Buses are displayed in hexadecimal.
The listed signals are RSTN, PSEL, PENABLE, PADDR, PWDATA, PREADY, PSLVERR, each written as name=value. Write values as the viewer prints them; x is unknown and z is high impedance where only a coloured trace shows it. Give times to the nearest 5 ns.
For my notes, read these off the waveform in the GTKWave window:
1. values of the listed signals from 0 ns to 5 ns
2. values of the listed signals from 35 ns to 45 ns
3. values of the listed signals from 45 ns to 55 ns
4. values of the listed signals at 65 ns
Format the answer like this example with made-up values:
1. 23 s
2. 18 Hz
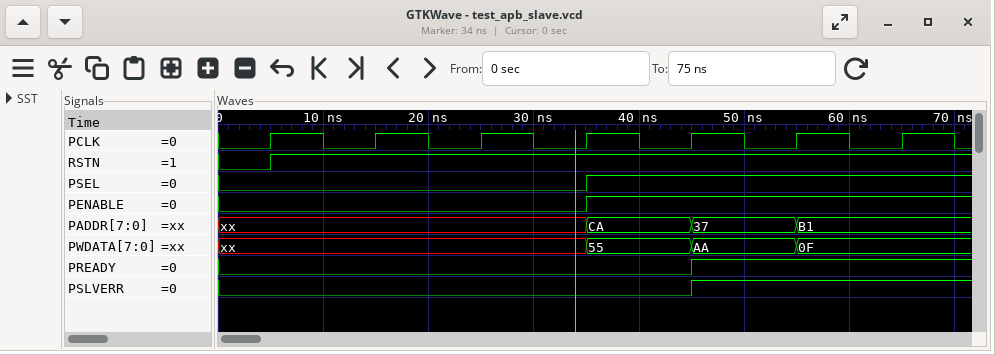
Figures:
1. RSTN=0, PSEL=0, PENABLE=0, PADDR=xx, PWDATA=xx, PREADY=0, PSLVERR=0
2. RSTN=1, PSEL=1, PENABLE=1, PADDR=CA, PWDATA=55, PREADY=0, PSLVERR=0
3. RSTN=1, PSEL=1, PENABLE=1, PADDR=37, PWDATA=AA, PREADY=1, PSLVERR=1
4. RSTN=1, PSEL=1, PENABLE=1, PADDR=B1, PWDATA=0F, PREADY=1, PSLVERR=1
